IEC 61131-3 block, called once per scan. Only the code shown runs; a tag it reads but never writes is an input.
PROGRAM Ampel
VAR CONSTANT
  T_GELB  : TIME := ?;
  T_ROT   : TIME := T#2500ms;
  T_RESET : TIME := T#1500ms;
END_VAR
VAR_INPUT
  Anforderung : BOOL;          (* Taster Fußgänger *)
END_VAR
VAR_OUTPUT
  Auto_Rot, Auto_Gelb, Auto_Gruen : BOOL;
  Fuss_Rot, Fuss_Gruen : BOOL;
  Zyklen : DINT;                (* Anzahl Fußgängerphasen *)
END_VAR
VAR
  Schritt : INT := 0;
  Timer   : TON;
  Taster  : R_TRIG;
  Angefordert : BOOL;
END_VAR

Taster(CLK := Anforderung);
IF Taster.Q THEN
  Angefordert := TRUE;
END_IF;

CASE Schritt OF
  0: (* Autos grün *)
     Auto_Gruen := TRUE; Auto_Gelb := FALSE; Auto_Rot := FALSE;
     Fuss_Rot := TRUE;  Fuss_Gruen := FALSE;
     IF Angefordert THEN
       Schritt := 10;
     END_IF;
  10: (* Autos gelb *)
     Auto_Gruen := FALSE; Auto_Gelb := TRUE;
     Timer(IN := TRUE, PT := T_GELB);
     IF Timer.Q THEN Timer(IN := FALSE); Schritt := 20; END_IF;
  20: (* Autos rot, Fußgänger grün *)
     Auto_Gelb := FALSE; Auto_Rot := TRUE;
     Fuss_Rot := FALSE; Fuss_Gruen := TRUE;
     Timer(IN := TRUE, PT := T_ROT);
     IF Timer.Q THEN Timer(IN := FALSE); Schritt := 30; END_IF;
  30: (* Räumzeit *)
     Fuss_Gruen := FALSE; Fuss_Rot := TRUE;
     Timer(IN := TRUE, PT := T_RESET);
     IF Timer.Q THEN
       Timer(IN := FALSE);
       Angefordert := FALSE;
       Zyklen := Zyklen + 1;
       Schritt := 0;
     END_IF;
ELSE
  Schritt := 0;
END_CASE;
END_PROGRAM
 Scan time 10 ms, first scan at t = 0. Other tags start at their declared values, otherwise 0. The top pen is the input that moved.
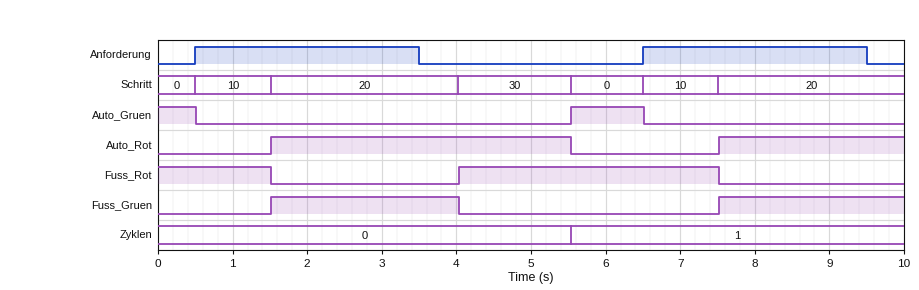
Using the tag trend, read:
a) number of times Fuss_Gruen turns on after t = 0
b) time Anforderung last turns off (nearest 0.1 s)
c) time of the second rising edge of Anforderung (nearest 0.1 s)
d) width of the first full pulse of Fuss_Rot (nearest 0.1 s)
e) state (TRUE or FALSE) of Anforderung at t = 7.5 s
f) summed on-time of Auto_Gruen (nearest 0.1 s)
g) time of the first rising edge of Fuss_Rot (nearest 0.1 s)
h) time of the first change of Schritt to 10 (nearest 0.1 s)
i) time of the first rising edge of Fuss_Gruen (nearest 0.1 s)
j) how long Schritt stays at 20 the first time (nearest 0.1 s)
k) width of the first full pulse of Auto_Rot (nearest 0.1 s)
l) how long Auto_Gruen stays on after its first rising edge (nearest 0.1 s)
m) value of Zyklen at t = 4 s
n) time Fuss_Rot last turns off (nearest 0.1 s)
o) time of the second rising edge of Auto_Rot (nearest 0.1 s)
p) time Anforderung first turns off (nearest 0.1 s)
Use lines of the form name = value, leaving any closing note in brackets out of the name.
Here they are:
number of times Fuss_Gruen turns on after t = 0 = 2
time Anforderung last turns off = 9.5 s
time of the second rising edge of Anforderung = 6.5 s
width of the first full pulse of Fuss_Rot = 3.5 s
state (TRUE or FALSE) of Anforderung at t = 7.5 s = TRUE
summed on-time of Auto_Gruen = 1.5 s
time of the first rising edge of Fuss_Rot = 4.0 s
time of the first change of Schritt to 10 = 0.5 s
time of the first rising edge of Fuss_Gruen = 1.5 s
how long Schritt stays at 20 the first time = 2.5 s
width of the first full pulse of Auto_Rot = 4.0 s
how long Auto_Gruen stays on after its first rising edge = 1.0 s
value of Zyklen at t = 4 s = 0
time Fuss_Rot last turns off = 7.5 s
time of the second rising edge of Auto_Rot = 7.5 s
time Anforderung first turns off = 3.5 s
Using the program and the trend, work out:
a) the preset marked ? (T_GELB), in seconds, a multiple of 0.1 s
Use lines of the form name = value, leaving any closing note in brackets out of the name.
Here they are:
the preset marked ? (T_GELB), in seconds, a multiple of 0.1 s = 1.0 s
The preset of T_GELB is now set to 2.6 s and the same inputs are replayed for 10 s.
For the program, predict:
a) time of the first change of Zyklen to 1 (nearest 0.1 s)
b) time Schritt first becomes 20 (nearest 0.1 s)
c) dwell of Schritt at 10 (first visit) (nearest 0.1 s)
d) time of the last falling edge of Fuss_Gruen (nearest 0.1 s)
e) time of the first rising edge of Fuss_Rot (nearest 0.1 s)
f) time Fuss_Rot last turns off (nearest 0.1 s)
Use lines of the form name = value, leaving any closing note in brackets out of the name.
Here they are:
time of the first change of Zyklen to 1 = 7.1 s
time Schritt first becomes 20 = 3.1 s
dwell of Schritt at 10 (first visit) = 2.6 s
time of the last falling edge of Fuss_Gruen = 5.6 s
time of the first rising edge of Fuss_Rot = 5.6 s
time Fuss_Rot last turns off = 3.1 s
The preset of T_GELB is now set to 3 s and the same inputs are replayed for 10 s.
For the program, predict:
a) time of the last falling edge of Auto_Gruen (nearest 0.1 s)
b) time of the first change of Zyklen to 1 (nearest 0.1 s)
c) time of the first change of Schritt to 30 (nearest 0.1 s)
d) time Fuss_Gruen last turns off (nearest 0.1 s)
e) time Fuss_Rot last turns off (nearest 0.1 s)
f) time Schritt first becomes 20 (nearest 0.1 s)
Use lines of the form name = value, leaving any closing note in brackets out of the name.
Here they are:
time of the last falling edge of Auto_Gruen = 0.5 s
time of the first change of Zyklen to 1 = 7.5 s
time of the first change of Schritt to 30 = 6.0 s
time Fuss_Gruen last turns off = 6.0 s
time Fuss_Rot last turns off = 3.5 s
time Schritt first becomes 20 = 3.5 s
